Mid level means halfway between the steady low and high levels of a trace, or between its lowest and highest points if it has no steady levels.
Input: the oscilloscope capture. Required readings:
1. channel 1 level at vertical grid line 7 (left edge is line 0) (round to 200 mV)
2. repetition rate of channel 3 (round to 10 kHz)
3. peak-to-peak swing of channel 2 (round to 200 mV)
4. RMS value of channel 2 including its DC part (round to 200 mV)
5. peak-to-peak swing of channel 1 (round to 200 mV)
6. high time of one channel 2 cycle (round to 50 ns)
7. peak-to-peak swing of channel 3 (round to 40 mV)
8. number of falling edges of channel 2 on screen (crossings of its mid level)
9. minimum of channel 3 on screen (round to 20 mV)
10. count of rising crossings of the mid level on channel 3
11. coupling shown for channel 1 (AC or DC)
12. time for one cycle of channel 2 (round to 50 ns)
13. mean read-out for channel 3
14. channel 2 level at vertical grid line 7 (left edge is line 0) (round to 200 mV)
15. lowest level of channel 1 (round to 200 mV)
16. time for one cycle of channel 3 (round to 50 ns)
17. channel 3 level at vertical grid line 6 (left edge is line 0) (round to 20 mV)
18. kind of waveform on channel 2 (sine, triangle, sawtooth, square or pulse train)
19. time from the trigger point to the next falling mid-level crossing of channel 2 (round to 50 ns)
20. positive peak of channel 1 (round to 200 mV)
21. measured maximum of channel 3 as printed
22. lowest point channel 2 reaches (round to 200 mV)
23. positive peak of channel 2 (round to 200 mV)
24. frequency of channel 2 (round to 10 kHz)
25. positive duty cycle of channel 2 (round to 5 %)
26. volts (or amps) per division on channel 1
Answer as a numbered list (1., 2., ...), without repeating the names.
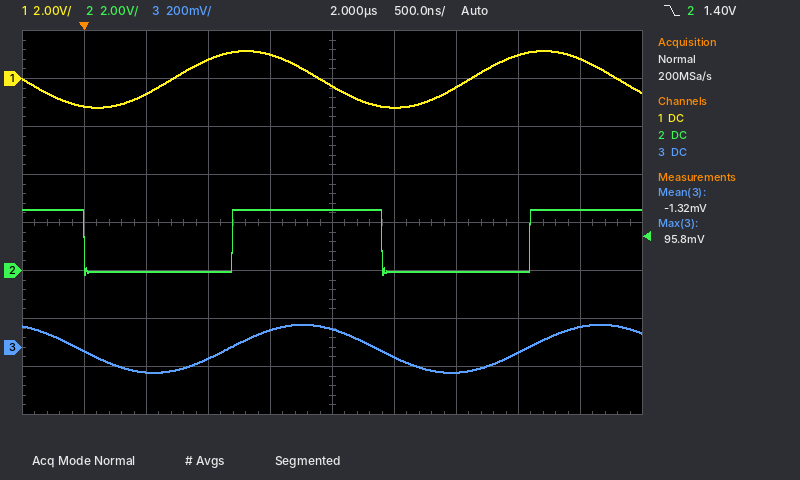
1. -400 mV
2. 420 kHz
3. 2.8 V
4. 1.8 V
5. 2.4 V
6. 1.20 µs
7. 200 mV
8. 2
9. -100 mV
10. 2
11. DC
12. 2.40 µs
13. -1.32 mV
14. 0.0 V
15. -1.2 V
16. 2.40 µs
17. -40 mV
18. square
19. 2.40 µs
20. 1.2 V
21. 95.8 mV
22. -200 mV
23. 2.6 V
24. 420 kHz
25. 50 %
26. 2 V
